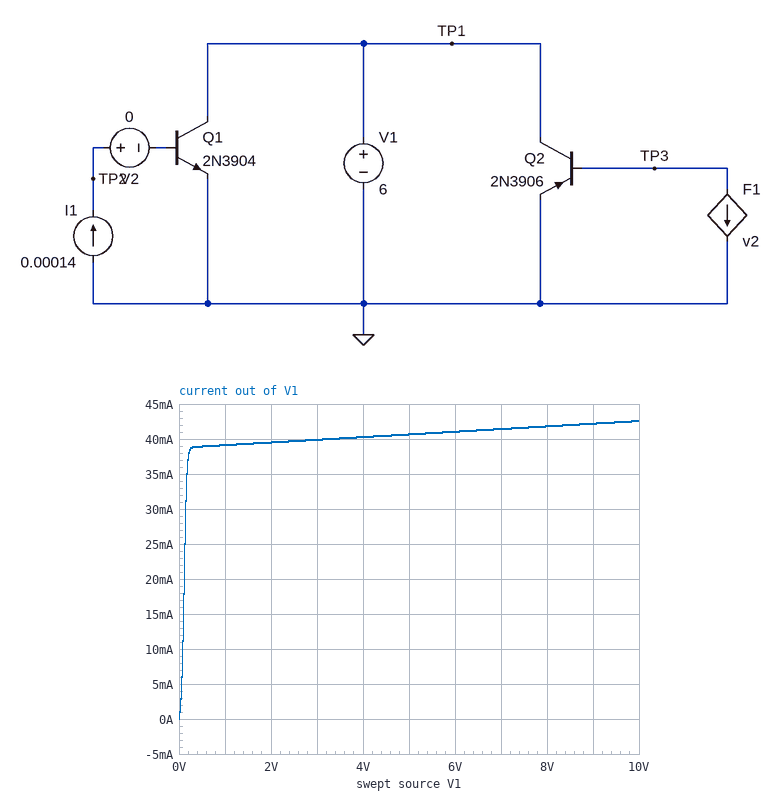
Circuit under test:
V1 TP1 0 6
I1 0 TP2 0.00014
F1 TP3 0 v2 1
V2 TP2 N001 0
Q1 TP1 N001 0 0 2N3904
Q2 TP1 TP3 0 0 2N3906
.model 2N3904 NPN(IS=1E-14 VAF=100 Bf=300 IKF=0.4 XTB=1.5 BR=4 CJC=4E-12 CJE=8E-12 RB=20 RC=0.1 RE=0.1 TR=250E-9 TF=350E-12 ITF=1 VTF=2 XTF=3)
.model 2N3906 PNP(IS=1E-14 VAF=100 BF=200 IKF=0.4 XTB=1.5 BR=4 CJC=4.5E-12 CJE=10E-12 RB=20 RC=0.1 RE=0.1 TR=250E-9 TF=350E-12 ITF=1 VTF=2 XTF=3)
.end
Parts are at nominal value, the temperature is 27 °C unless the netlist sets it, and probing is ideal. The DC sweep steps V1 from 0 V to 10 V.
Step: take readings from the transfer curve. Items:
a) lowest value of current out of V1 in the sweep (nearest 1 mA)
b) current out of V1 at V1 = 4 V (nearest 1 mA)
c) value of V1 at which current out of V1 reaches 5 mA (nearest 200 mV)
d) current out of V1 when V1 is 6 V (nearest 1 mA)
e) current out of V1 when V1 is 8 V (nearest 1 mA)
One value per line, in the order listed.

0 A
40 mA
0 V
41 mA
42 mA
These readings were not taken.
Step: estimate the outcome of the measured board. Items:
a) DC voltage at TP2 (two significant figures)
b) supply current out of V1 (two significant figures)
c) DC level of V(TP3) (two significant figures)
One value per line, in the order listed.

760 mV
41 mA
5.4 V
